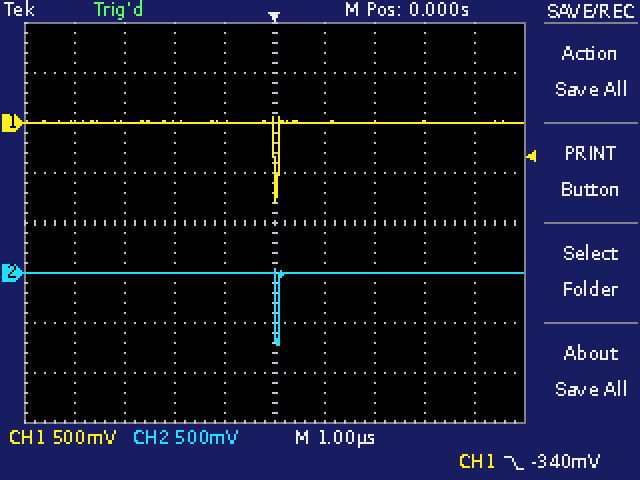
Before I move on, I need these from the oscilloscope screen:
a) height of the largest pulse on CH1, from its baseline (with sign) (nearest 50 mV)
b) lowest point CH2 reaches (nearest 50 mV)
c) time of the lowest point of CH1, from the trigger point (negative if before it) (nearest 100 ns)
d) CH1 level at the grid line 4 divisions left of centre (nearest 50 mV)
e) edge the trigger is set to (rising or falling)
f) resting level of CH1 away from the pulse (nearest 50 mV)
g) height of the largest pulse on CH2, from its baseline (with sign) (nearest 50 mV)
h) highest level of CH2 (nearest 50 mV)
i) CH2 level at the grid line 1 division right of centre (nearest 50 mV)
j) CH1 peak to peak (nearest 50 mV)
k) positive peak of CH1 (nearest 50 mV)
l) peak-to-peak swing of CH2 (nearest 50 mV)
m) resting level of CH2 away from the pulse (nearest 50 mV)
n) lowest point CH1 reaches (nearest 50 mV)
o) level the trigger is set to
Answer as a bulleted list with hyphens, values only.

- -800 mV
- -700 mV
- 0.0 µs
- 0 mV
- falling
- 0 mV
- -700 mV
- 50 mV
- 0 mV
- 850 mV
- 50 mV
- 750 mV
- 0 mV
- -800 mV
- -340 mV
